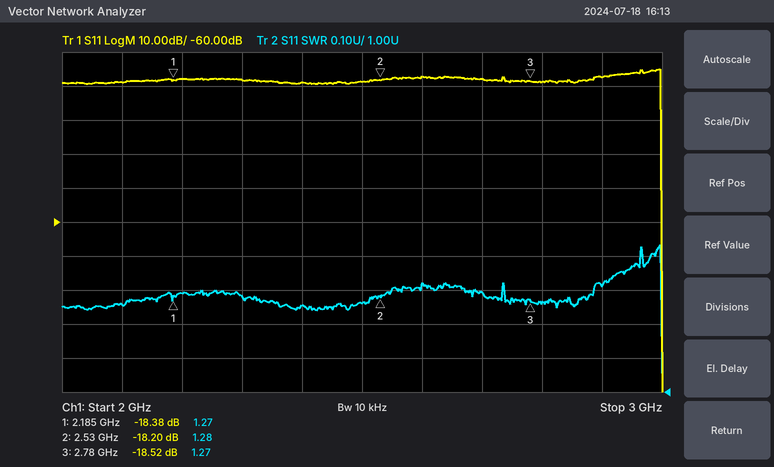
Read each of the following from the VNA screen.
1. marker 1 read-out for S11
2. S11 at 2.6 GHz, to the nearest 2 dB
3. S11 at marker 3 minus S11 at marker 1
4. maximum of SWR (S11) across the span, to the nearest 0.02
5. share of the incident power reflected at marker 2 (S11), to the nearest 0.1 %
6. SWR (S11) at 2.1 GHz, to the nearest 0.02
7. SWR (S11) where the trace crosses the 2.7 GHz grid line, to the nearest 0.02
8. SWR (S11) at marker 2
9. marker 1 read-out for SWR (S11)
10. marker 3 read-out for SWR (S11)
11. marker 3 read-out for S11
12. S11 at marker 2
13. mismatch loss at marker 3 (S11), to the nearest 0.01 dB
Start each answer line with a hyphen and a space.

- -18.38 dB
- -18 dB
- -0.14 dB
- 1.44
- 1.5 %
- 1.26
- 1.30
- 1.28
- 1.27
- 1.27
- -18.52 dB
- -18.20 dB
- 0.06 dB
